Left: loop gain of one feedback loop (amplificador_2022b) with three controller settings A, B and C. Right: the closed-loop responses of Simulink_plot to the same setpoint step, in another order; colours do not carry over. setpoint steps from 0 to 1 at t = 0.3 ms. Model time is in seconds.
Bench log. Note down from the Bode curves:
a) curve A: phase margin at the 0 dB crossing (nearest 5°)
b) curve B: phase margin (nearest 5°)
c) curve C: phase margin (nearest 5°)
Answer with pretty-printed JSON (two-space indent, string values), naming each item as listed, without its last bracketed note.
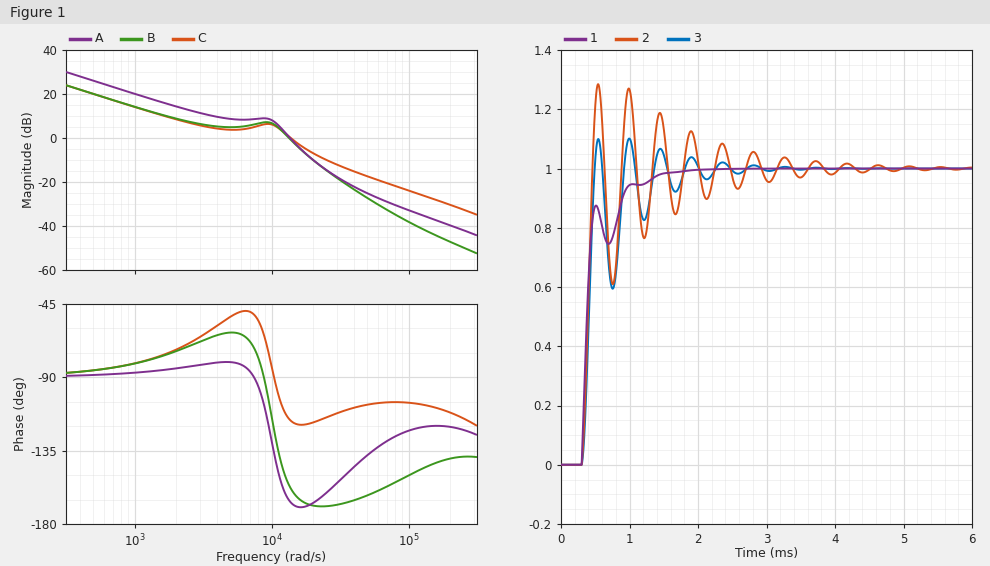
{
  "curve A: phase margin at the 0 dB crossing": "15°",
  "curve B: phase margin": "25°",
  "curve C: phase margin": "65°"
}
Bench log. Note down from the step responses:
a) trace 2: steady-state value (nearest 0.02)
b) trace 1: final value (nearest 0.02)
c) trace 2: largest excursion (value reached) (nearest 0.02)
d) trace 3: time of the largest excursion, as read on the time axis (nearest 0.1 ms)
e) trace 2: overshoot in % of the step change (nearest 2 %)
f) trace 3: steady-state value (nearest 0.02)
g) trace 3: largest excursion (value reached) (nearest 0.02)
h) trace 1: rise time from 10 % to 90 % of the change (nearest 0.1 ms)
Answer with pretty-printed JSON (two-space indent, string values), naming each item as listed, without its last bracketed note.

{
  "trace 2: steady-state value": "1.00",
  "trace 1: final value": "1.00",
  "trace 2: largest excursion (value reached)": "1.28",
  "trace 3: time of the largest excursion, as read on the time axis": "1.0 ms",
  "trace 2: overshoot in % of the step change": "28 %",
  "trace 3: steady-state value": "1.00",
  "trace 3: largest excursion (value reached)": "1.10",
  "trace 1: rise time from 10 % to 90 % of the change": "0.6 ms"
}
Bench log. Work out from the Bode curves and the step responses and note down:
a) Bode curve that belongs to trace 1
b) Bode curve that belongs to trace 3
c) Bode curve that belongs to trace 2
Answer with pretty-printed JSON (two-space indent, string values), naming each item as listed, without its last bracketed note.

{
  "Bode curve that belongs to trace 1": "C",
  "Bode curve that belongs to trace 3": "B",
  "Bode curve that belongs to trace 2": "A"
}
